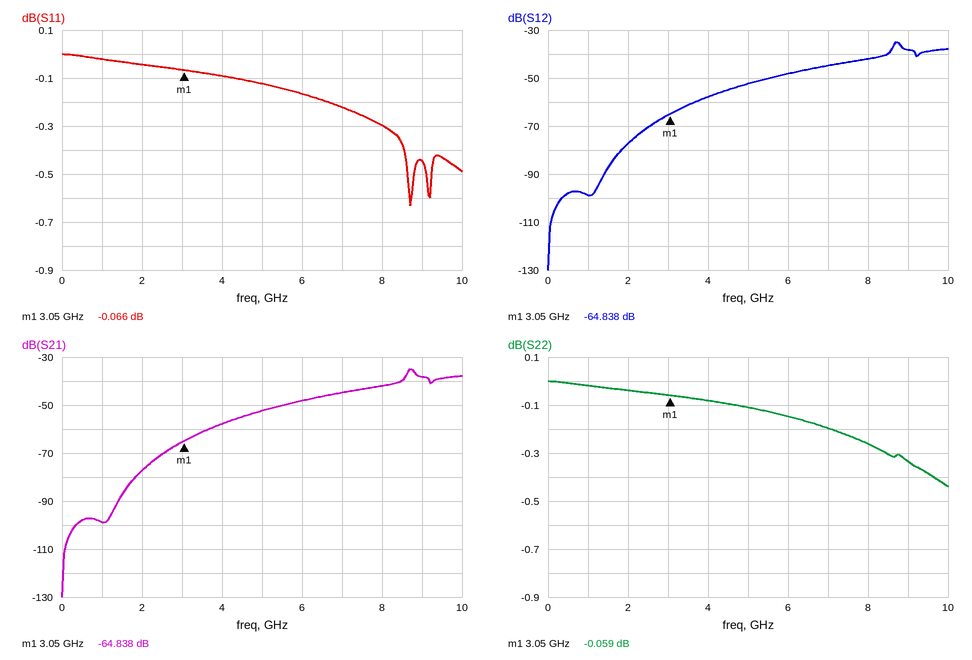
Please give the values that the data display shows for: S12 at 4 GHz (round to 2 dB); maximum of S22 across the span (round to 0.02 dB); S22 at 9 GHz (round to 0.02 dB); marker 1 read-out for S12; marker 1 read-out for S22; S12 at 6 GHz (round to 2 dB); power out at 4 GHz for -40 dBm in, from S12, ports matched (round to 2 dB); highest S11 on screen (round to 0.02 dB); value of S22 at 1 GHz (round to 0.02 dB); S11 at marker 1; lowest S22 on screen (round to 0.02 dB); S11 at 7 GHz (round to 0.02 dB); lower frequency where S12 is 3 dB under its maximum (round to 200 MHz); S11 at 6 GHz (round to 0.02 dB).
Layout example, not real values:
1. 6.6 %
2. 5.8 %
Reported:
1. -58 dB
2. 0.00 dB
3. -0.34 dB
4. -64.838 dB
5. -0.059 dB
6. -48 dB
7. -98 dBm
8. 0.00 dB
9. -0.02 dB
10. -0.066 dB
11. -0.44 dB
12. -0.22 dB
13. 8.6 GHz
14. -0.16 dB
